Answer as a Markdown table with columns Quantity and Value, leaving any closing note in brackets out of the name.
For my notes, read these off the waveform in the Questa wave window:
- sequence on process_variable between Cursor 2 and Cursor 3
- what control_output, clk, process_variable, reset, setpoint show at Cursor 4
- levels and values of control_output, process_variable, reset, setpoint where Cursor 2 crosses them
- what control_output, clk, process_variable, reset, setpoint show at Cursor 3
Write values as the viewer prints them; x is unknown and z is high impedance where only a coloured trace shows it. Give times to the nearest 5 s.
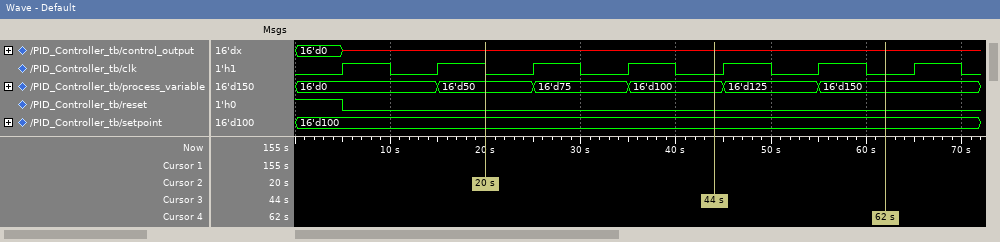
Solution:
| Quantity | Value |
|---|---|
| sequence on process_variable between Cursor 2 and Cursor 3 | 16'd50, 16'd75, 16'd100 |
| what control_output, clk, process_variable, reset, setpoint show at Cursor 4 | control_output=x, clk=0, process_variable=16'd150, reset=0, setpoint=16'd100 |
| levels and values of control_output, process_variable, reset, setpoint where Cursor 2 crosses them | control_output=x, process_variable=16'd50, reset=0, setpoint=16'd100 |
| what control_output, clk, process_variable, reset, setpoint show at Cursor 3 | control_output=x, clk=0, process_variable=16'd100, reset=0, setpoint=16'd100 |
